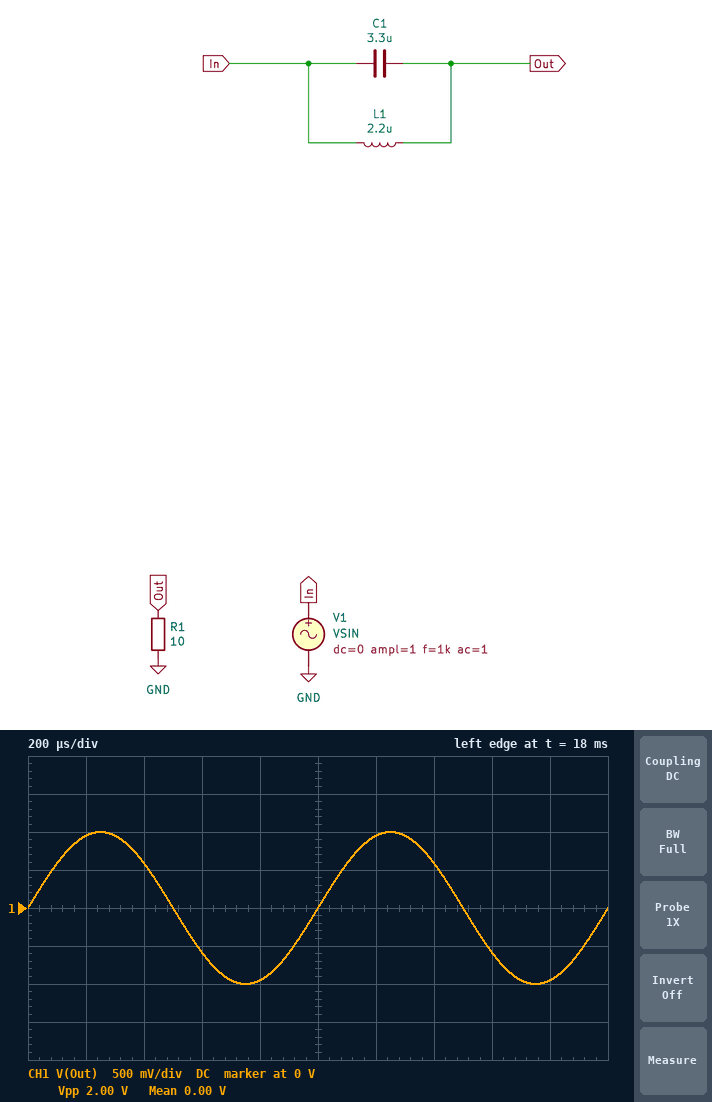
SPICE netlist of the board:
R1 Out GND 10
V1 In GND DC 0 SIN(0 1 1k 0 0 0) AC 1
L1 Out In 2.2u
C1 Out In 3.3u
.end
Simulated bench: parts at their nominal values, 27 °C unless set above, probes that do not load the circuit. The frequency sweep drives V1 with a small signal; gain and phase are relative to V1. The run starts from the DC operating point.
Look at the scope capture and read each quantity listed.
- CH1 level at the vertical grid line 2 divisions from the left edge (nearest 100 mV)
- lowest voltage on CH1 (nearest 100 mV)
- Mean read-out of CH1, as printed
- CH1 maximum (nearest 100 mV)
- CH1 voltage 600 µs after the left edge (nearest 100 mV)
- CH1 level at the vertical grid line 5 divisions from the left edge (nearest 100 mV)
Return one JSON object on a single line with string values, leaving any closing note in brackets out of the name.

{"CH1 level at the vertical grid line 2 divisions from the left edge": "600 mV", "lowest voltage on CH1": "-1.0 V", "Mean read-out of CH1, as printed": "0.00 V", "CH1 maximum": "1.0 V", "CH1 voltage 600 µs after the left edge": "-600 mV", "CH1 level at the vertical grid line 5 divisions from the left edge": "0 V"}
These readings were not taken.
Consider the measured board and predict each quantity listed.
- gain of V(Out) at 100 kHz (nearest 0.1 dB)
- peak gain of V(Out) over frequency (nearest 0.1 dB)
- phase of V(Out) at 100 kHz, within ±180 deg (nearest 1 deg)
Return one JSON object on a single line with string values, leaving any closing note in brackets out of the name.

{"gain of V(Out) at 100 kHz": "0 dB", "peak gain of V(Out) over frequency": "0 dB", "phase of V(Out) at 100 kHz, within ±180 deg": "4 deg"}
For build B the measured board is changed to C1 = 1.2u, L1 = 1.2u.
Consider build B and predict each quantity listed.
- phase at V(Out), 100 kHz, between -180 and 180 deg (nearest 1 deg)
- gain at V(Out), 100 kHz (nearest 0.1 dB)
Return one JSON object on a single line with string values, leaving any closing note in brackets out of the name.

{"phase at V(Out), 100 kHz, between -180 and 180 deg": "-10 deg", "gain at V(Out), 100 kHz": "-0.1 dB"}
